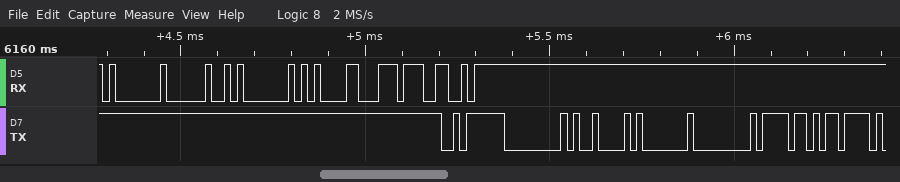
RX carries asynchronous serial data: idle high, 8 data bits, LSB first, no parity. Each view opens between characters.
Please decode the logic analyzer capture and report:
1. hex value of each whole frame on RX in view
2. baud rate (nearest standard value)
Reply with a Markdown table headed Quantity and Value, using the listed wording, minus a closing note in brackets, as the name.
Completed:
| Quantity | Value |
|---|---|
| hex value of each whole frame on RX in view | 01, 20, 01, 85, DC, A6 |
| baud rate | 57600 baud |
